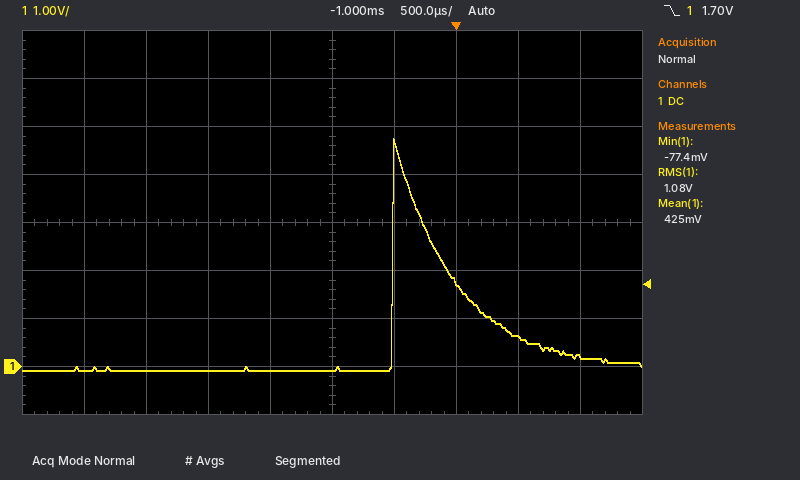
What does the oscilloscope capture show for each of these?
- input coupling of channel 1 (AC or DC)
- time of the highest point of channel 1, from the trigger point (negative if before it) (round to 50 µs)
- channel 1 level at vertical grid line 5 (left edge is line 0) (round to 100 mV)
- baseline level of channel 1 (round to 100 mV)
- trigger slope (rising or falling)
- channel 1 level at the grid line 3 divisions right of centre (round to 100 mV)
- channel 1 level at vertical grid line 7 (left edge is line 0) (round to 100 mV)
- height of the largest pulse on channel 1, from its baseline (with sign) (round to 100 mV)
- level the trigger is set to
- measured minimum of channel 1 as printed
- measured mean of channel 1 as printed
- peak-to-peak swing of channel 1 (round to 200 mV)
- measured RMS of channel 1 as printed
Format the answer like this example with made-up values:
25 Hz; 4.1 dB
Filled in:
DC; -500 µs; -100 mV; -100 mV; falling; 600 mV; 1.8 V; +4.8 V; 1.70 V; -77.4 mV; 425 mV; 4.8 V; 1.08 V
